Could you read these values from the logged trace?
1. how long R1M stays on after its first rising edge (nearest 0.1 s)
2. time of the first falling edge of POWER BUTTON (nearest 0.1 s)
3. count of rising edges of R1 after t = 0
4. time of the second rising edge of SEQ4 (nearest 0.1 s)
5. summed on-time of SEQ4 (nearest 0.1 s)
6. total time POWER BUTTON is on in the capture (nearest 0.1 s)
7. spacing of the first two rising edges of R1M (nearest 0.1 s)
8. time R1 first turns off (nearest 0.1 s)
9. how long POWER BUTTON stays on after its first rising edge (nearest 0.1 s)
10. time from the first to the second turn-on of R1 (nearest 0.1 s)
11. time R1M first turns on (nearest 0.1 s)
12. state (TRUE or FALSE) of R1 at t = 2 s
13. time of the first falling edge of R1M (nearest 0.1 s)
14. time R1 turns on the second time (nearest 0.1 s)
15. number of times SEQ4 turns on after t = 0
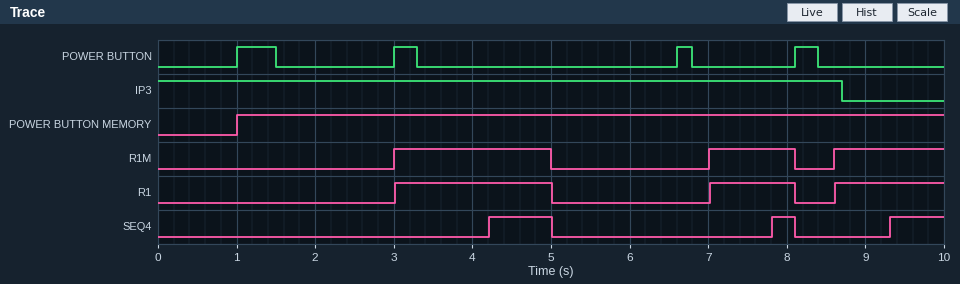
2.0 s
1.5 s
3
7.8 s
1.8 s
1.3 s
4.0 s
5.0 s
0.5 s
4.0 s
3.0 s
FALSE
5.0 s
7.0 s
3
